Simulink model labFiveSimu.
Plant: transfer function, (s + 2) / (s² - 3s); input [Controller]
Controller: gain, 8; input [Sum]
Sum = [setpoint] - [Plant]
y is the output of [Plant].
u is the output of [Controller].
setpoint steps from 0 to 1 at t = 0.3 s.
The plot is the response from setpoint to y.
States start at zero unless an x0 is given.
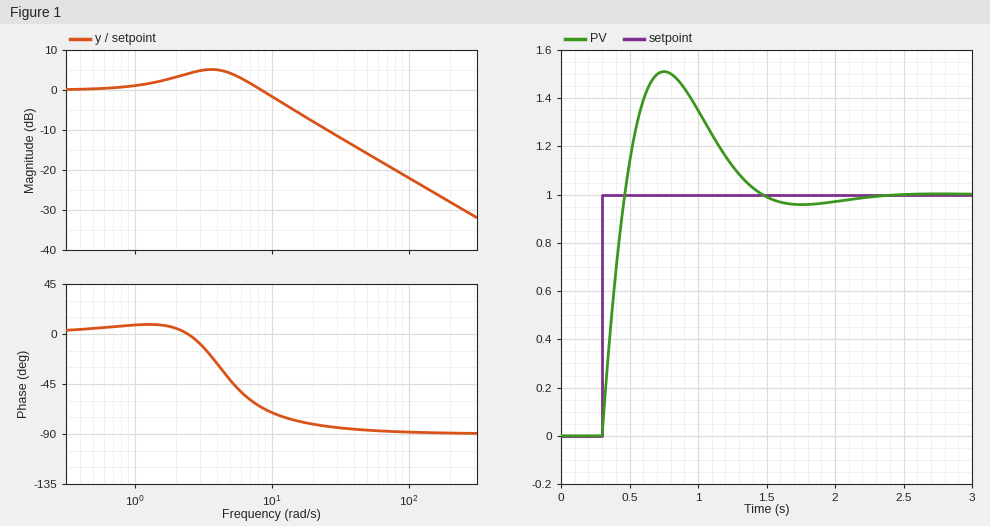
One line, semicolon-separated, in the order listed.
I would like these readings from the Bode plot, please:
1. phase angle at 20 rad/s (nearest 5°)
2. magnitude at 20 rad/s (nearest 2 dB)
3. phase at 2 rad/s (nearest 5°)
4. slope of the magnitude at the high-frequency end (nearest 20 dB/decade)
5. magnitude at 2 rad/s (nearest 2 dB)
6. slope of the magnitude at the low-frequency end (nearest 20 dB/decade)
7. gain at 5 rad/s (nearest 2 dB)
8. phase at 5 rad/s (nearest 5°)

-80°; -8 dB; 5°; -20 dB/decade; 4 dB; 0 dB/decade; 4 dB; -40°
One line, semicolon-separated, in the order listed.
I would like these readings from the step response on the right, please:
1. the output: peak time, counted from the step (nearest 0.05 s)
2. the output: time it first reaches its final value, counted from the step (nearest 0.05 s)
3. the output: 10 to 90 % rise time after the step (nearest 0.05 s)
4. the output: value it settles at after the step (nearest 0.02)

0.45 s; 0.15 s; 0.15 s; 1.00
